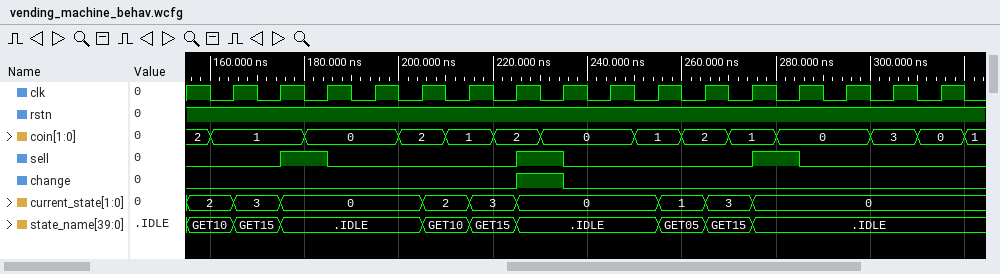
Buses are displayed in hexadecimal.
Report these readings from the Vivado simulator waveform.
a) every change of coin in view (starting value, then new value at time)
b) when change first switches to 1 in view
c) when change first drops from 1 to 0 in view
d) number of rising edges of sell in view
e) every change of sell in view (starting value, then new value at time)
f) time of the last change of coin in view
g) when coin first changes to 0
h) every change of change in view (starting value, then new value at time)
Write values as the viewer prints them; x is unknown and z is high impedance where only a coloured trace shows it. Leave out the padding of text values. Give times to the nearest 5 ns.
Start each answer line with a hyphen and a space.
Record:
- 2, 1 at 160 ns, 0 at 180 ns, 2 at 200 ns, 1 at 210 ns, 2 at 220 ns, 0 at 230 ns, 1 at 250 ns, 2 at 260 ns, 1 at 270 ns, 0 at 280 ns, 3 at 300 ns, 0 at 310 ns, 1 at 320 ns
- 225 ns
- 235 ns
- 3
- 0, 1 at 175 ns, 0 at 185 ns, 1 at 225 ns, 0 at 235 ns, 1 at 275 ns, 0 at 285 ns
- 320 ns
- 180 ns
- 0, 1 at 225 ns, 0 at 235 ns
